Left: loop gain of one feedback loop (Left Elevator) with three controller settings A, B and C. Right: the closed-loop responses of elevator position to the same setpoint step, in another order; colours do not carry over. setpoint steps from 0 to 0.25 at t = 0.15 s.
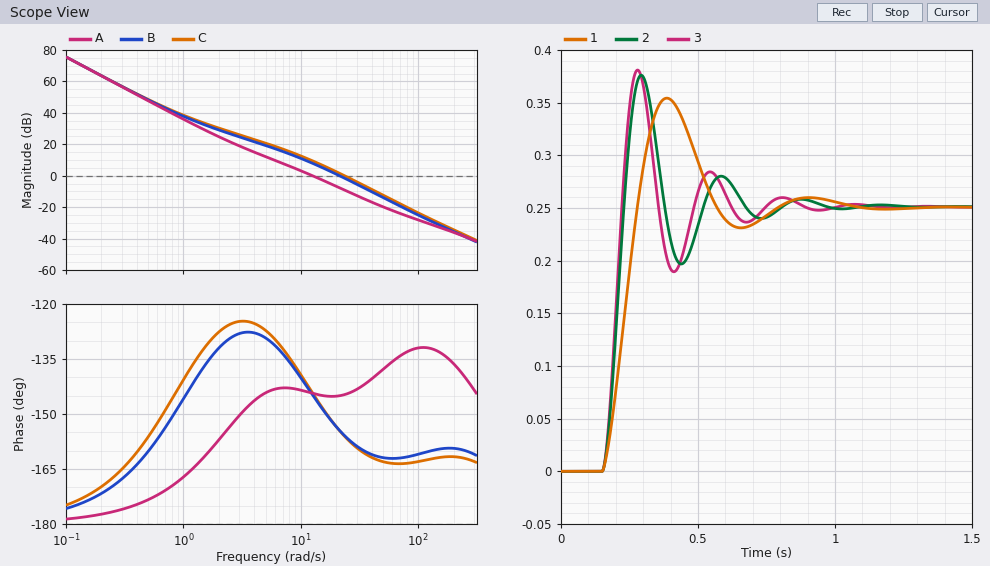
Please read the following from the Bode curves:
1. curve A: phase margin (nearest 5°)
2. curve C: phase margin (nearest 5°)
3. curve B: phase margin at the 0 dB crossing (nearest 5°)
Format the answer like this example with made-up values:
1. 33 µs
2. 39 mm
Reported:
1. 35°
2. 25°
3. 25°
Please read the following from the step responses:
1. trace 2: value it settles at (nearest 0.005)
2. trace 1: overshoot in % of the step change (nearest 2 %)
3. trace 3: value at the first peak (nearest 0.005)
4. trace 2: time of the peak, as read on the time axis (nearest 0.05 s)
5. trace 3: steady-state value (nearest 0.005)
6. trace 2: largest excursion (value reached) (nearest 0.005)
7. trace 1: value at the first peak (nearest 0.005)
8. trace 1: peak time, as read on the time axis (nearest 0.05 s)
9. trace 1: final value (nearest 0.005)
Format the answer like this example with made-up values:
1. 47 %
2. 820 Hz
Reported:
1. 0.250
2. 42 %
3. 0.380
4. 0.30 s
5. 0.250
6. 0.375
7. 0.355
8. 0.40 s
9. 0.250
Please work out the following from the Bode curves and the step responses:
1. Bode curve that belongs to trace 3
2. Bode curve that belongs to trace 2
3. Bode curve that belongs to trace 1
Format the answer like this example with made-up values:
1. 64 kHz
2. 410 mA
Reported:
1. C
2. B
3. A
